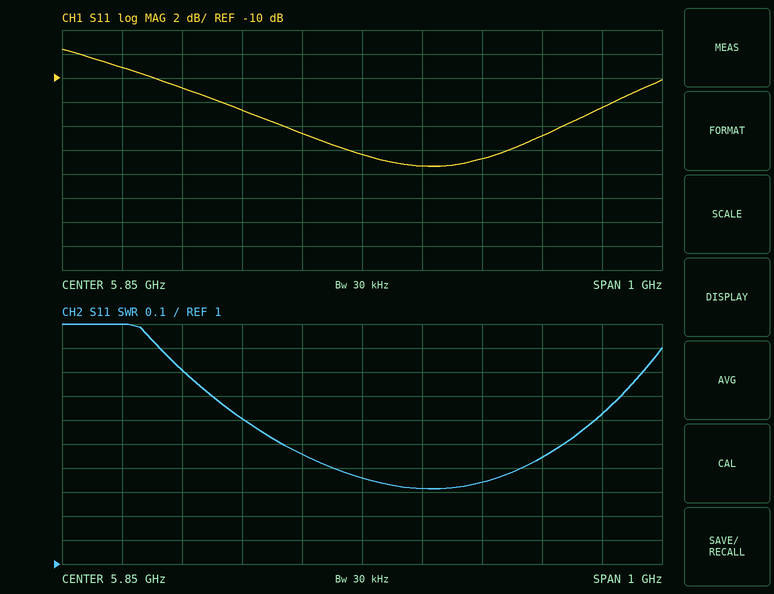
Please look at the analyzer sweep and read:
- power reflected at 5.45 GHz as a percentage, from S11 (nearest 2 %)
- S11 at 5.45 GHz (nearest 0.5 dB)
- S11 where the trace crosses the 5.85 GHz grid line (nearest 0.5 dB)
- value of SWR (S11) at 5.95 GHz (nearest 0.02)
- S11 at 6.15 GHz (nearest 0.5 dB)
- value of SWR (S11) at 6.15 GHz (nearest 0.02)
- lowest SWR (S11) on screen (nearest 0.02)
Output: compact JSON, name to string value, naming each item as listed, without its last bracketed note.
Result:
{"power reflected at 5.45 GHz as a percentage, from S11": "12 %", "S11 at 5.45 GHz": "-9.0 dB", "S11 where the trace crosses the 5.85 GHz grid line": "-16.5 dB", "value of SWR (S11) at 5.95 GHz": "1.32", "S11 at 6.15 GHz": "-15.0 dB", "value of SWR (S11) at 6.15 GHz": "1.44", "lowest SWR (S11) on screen": "1.32"}
